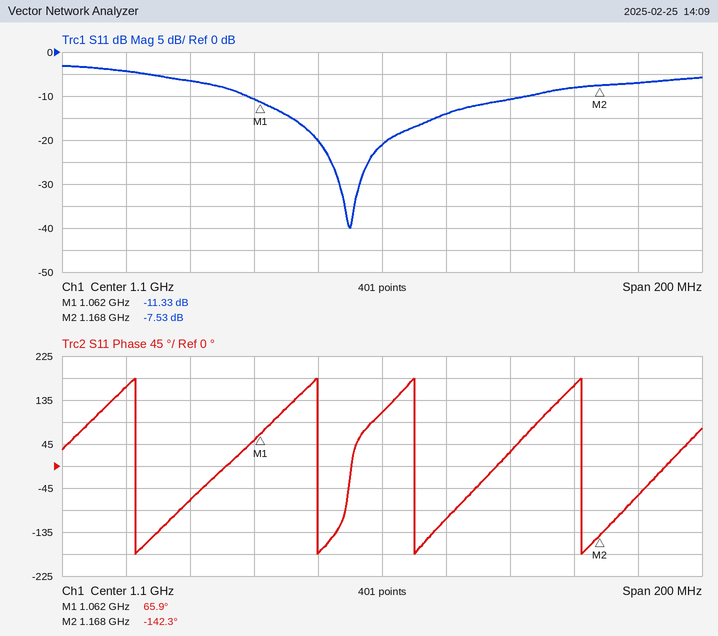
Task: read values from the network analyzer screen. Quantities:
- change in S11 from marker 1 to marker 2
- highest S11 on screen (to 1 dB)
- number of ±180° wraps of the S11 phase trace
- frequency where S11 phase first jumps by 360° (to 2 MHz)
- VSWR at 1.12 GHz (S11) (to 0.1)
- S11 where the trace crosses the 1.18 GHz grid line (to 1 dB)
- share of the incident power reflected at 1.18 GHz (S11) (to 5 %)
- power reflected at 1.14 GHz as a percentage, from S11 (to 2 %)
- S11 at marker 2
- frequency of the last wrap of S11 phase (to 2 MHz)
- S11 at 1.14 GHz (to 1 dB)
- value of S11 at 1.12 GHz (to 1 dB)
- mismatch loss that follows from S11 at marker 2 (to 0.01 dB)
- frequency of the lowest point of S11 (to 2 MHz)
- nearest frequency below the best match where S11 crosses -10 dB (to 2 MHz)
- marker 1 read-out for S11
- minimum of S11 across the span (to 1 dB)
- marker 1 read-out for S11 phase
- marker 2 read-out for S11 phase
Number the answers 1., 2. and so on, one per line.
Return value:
1. 3.80 dB
2. -3 dB
3. 4
4. 1.022 GHz
5. 1.5
6. -7 dB
7. 20 %
8. 8 %
9. -7.53 dB
10. 1.162 GHz
11. -11 dB
12. -14 dB
13. 0.84 dB
14. 1.090 GHz
15. 1.058 GHz
16. -11.33 dB
17. -40 dB
18. 65.9°
19. -142.3°
